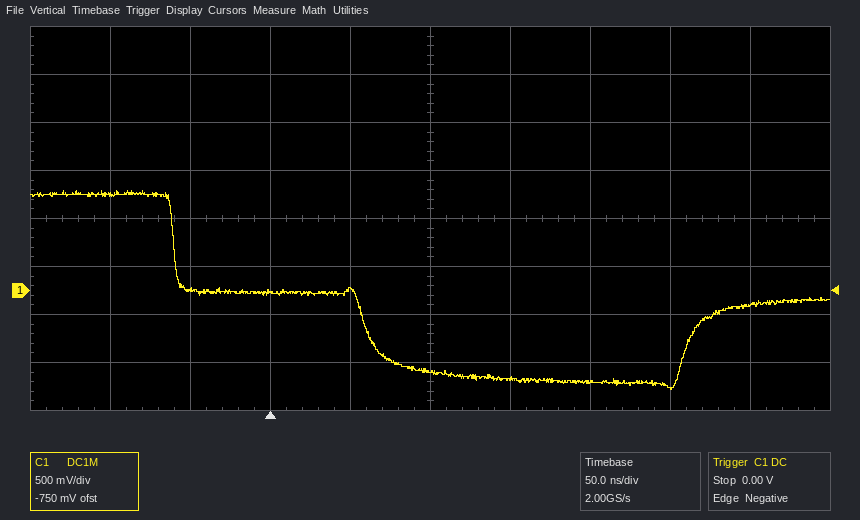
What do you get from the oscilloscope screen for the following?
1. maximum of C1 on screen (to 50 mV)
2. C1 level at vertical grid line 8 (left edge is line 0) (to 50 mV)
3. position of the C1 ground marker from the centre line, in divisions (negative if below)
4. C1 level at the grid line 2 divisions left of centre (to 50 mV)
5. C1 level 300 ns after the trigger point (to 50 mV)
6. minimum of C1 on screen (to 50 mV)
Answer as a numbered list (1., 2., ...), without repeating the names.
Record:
1. 1.05 V
2. -1.00 V
3. -1.5 div
4. 0 mV
5. -150 mV
6. -1.05 V
